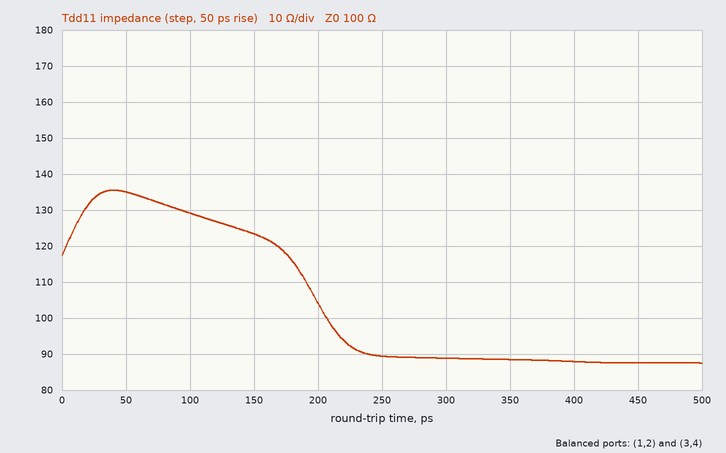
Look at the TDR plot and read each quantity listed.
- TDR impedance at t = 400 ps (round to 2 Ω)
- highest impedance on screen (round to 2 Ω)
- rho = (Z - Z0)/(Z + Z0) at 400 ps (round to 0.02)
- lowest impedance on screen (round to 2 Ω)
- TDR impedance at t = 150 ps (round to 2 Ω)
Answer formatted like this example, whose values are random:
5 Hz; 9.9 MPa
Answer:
88 Ω; 136 Ω; -0.06; 88 Ω; 124 Ω
